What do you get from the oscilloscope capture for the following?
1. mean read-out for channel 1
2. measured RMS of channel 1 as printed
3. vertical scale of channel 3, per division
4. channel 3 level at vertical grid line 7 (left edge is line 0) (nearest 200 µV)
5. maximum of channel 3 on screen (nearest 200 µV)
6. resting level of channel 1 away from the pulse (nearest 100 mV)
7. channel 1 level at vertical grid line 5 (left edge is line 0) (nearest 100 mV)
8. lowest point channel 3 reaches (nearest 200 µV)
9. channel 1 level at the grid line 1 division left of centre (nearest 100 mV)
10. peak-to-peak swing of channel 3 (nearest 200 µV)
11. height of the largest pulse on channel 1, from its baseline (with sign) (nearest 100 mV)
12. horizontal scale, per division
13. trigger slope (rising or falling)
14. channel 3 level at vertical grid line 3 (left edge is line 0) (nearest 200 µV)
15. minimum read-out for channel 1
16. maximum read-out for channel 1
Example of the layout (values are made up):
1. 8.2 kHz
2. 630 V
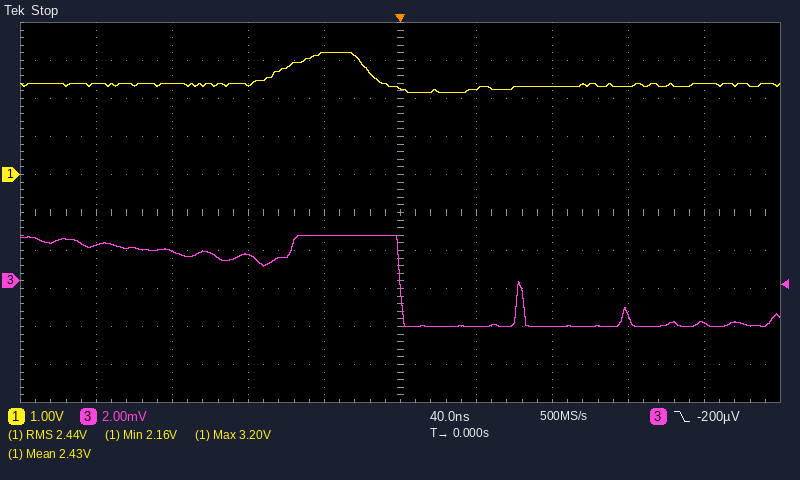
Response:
1. 2.43 V
2. 2.44 V
3. 2 mV
4. -2.4 mV
5. 2.4 mV
6. 2.4 V
7. 2.3 V
8. -2.4 mV
9. 3.2 V
10. 4.8 mV
11. +800 mV
12. 40 ns
13. falling
14. 1.4 mV
15. 2.16 V
16. 3.20 V
